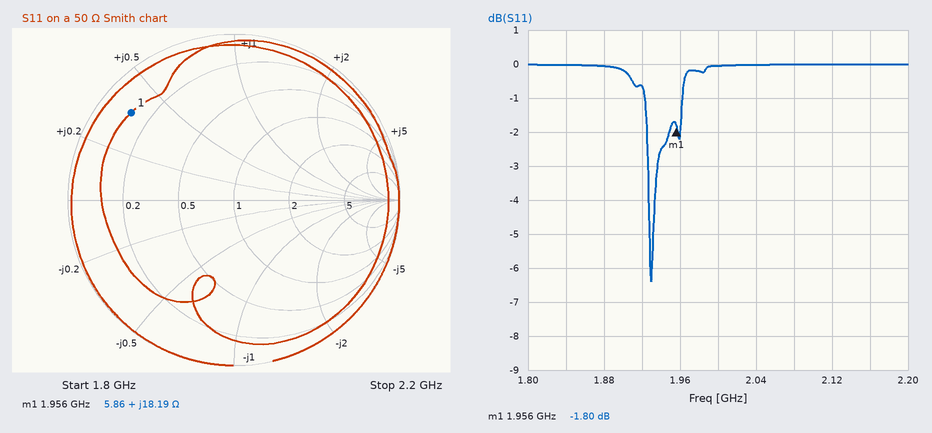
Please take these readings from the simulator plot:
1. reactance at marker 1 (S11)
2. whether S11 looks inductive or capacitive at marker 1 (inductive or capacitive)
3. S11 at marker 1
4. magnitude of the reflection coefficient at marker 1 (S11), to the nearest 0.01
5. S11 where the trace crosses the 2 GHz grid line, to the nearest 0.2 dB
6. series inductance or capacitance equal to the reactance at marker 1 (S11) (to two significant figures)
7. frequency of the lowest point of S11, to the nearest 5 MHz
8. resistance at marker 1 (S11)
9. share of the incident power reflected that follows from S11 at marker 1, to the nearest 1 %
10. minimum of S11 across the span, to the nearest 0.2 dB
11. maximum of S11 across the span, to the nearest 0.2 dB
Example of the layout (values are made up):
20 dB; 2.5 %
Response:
+18.19 Ω; inductive; -1.80 dB; 0.81; 0.0 dB; 1.5 nH; 1.930 GHz; 5.86 Ω; 66 %; -6.4 dB; 0.0 dB
